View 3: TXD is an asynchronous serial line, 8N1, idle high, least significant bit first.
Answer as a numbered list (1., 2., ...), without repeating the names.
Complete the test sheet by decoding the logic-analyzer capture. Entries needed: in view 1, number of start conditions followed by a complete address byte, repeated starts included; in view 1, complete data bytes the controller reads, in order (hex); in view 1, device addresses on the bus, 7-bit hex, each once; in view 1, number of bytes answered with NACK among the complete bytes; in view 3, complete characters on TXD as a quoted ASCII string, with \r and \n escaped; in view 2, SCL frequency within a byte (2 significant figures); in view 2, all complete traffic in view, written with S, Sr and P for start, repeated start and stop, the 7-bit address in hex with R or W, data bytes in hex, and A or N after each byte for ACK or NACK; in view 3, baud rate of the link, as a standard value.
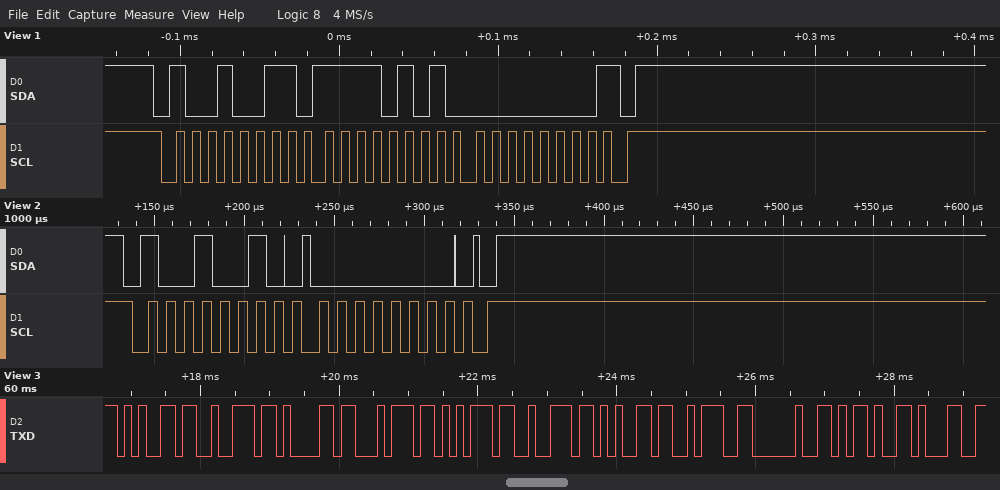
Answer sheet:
1. 1
2. F5 00
3. 0x49
4. 1
5. "erature: -1"
6. 100 kHz
7. S 49W A 00 A P
8. 9600 baud
